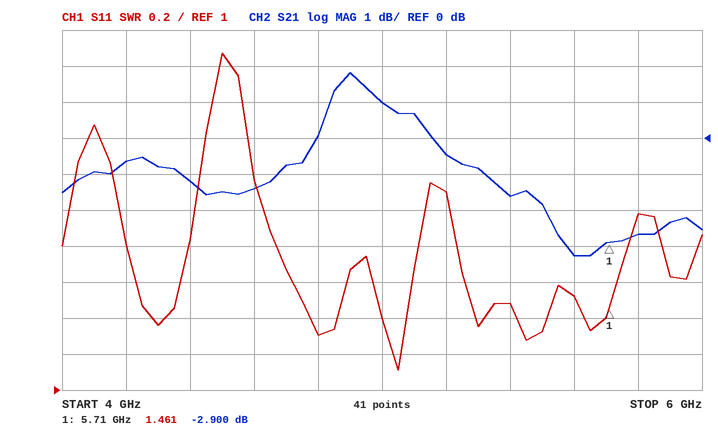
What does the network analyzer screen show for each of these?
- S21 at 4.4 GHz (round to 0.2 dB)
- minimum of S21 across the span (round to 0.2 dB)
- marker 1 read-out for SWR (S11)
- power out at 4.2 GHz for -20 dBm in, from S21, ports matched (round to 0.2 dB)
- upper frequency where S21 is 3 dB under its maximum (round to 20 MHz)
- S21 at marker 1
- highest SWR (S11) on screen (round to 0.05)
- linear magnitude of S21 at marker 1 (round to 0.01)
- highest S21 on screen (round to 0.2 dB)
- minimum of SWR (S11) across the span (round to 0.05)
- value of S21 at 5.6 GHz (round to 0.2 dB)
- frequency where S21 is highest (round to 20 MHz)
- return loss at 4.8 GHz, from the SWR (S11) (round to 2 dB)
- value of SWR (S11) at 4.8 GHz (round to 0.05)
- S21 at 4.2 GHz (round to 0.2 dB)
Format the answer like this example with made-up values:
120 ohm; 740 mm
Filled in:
-1.2 dB; -3.2 dB; 1.461; -20.6 dBm; 5.34 GHz; -2.900 dB; 2.85; 0.72; 1.8 dB; 1.10; -3.2 dB; 4.90 GHz; 18 dB; 1.30; -0.6 dB
